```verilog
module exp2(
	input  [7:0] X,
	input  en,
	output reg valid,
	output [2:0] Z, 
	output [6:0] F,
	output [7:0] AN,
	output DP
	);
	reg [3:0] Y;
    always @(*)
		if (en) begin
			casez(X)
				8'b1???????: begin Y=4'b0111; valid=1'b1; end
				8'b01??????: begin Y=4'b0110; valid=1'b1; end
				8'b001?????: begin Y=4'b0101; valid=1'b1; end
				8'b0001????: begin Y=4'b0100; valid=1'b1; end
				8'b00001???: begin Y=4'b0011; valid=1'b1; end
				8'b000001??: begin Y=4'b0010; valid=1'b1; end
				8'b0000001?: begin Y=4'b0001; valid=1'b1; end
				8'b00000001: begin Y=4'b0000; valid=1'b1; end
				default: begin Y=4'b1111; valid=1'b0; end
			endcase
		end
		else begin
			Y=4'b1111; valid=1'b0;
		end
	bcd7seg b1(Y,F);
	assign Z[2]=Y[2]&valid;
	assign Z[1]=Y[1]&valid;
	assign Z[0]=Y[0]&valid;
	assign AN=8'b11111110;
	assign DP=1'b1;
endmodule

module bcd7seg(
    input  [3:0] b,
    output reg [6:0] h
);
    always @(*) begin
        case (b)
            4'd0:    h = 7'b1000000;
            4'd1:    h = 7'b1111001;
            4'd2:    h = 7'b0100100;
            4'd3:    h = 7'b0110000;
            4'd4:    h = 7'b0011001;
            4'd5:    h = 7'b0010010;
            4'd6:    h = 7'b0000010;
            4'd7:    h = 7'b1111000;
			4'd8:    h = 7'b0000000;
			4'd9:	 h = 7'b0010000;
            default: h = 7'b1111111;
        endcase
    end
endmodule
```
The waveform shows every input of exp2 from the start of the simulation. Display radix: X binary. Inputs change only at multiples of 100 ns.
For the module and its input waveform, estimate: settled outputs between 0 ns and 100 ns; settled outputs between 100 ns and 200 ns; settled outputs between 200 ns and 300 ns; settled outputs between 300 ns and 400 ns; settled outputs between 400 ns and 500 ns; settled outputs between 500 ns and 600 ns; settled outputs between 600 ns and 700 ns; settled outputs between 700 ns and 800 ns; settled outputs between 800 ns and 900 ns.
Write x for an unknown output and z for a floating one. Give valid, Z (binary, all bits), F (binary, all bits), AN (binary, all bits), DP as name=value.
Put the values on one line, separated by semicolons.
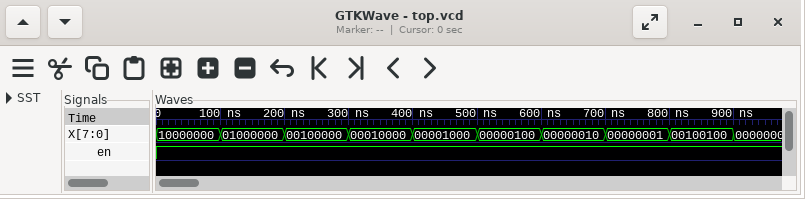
valid=1, Z=111, F=1111000, AN=11111110, DP=1; valid=1, Z=110, F=0000010, AN=11111110, DP=1; valid=1, Z=101, F=0010010, AN=11111110, DP=1; valid=1, Z=100, F=0011001, AN=11111110, DP=1; valid=1, Z=011, F=0110000, AN=11111110, DP=1; valid=1, Z=010, F=0100100, AN=11111110, DP=1; valid=1, Z=001, F=1111001, AN=11111110, DP=1; valid=1, Z=000, F=1000000, AN=11111110, DP=1; valid=1, Z=101, F=0010010, AN=11111110, DP=1
